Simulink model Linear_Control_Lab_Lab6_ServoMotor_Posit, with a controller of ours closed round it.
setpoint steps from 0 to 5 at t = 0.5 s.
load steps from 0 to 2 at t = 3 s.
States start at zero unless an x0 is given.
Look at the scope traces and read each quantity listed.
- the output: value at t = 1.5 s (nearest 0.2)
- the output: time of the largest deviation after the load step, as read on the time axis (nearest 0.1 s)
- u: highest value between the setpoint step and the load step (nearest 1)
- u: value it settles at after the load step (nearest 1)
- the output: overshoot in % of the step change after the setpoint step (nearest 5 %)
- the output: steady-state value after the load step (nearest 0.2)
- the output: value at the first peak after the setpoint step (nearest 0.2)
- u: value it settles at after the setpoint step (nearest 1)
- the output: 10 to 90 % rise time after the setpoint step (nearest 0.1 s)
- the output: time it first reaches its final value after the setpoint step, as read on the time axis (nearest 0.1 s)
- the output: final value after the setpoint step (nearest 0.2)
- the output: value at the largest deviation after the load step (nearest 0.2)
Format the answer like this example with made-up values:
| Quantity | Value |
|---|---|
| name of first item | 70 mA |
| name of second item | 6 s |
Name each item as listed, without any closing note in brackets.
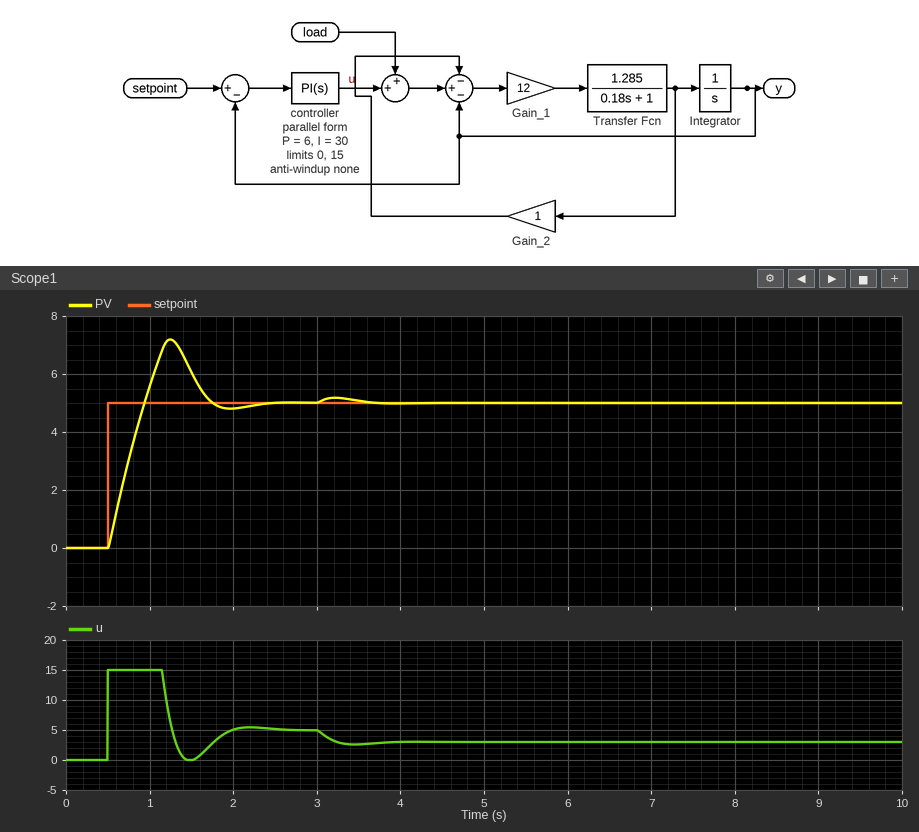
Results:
| Quantity | Value |
|---|---|
| the output: value at t = 1.5 s | 6.0 |
| the output: time of the largest deviation after the load step, as read on the time axis | 3.2 s |
| u: highest value between the setpoint step and the load step | 15 |
| u: value it settles at after the load step | 3 |
| the output: overshoot in % of the step change after the setpoint step | 45 % |
| the output: steady-state value after the load step | 5.0 |
| the output: value at the first peak after the setpoint step | 7.2 |
| u: value it settles at after the setpoint step | 5 |
| the output: 10 to 90 % rise time after the setpoint step | 0.3 s |
| the output: time it first reaches its final value after the setpoint step, as read on the time axis | 0.9 s |
| the output: final value after the setpoint step | 5.0 |
| the output: value at the largest deviation after the load step | 5.2 |
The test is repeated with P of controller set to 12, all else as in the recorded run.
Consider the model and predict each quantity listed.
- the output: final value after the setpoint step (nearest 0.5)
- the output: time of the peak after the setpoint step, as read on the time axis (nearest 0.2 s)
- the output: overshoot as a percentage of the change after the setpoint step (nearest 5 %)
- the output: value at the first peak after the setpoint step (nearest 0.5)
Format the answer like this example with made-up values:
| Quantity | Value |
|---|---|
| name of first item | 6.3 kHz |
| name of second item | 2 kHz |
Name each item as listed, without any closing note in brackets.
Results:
| Quantity | Value |
|---|---|
| the output: final value after the setpoint step | 5.0 |
| the output: time of the peak after the setpoint step, as read on the time axis | 1.2 s |
| the output: overshoot as a percentage of the change after the setpoint step | 30 % |
| the output: value at the first peak after the setpoint step | 6.5 |
